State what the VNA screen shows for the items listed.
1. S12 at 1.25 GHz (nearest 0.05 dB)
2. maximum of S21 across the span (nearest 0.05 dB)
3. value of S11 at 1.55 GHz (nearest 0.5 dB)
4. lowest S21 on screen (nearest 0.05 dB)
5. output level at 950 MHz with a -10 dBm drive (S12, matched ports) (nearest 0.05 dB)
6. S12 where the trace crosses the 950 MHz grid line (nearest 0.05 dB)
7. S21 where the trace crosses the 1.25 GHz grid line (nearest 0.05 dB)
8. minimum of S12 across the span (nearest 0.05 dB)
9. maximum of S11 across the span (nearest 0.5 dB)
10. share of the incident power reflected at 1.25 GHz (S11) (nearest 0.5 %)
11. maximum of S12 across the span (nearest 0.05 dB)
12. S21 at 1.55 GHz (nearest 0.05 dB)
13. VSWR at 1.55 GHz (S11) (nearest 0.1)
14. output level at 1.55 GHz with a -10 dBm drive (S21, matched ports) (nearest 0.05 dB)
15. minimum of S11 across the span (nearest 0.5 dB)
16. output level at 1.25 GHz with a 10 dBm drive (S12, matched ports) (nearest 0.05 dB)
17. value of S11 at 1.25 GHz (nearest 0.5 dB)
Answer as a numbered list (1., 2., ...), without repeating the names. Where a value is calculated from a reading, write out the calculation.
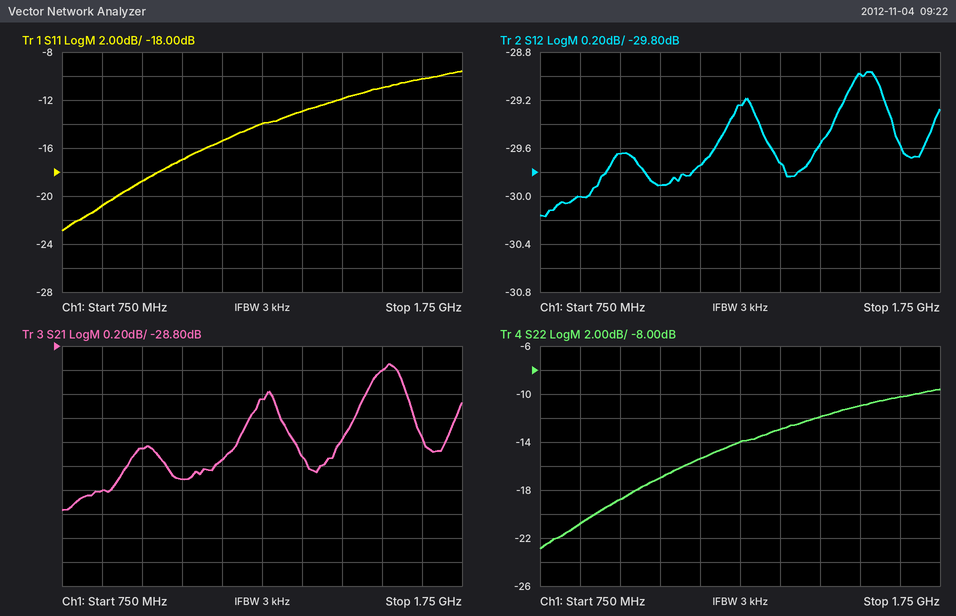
1. -29.25 dB
2. -28.95 dB
3. -11.0 dB
4. -30.15 dB
5. -10 dBm + (-29.65 dB) = -39.65 dBm
6. -29.65 dB
7. -29.25 dB
8. -30.15 dB
9. -9.5 dB
10. 10^(-14/10) ≈ 4.0 %
11. -28.95 dB
12. -29.00 dB
13. |Γ| = 10^(-11/20) = 0.2818; VSWR = (1 + 0.2818)/(1 − 0.2818) ≈ 1.8
14. -10 dBm + (-29.00 dB) = -39.00 dBm
15. -23.0 dB
16. 10 dBm + (-29.25 dB) = -19.25 dBm
17. -14.0 dB
